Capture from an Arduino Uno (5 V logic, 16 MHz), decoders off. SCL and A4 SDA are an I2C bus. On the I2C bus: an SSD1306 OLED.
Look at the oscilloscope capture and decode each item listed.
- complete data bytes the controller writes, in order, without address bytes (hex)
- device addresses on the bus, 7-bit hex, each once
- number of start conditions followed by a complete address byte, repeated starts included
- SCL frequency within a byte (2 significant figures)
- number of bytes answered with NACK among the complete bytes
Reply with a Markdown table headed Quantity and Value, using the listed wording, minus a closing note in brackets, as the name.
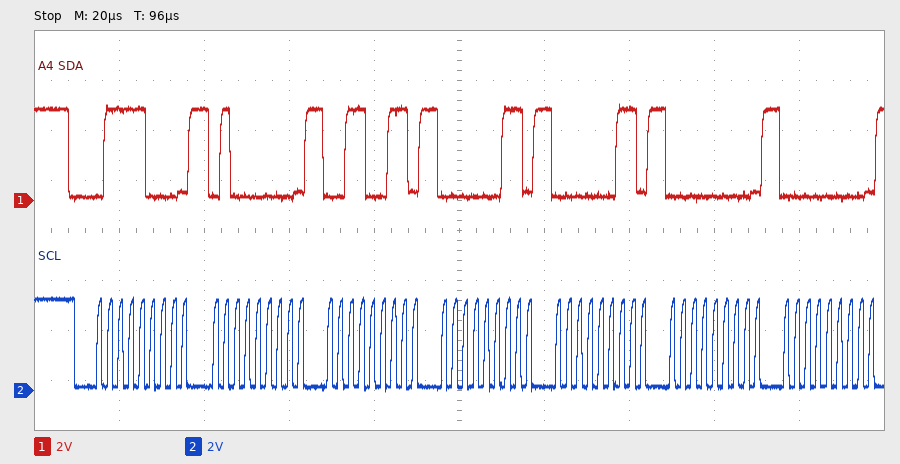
| Quantity | Value |
|---|---|
| complete data bytes the controller writes, in order, without address bytes | 40 33 03 03 00 00 |
| device addresses on the bus, 7-bit hex, each once | 0x3C |
| number of start conditions followed by a complete address byte, repeated starts included | 1 |
| SCL frequency within a byte | 400 kHz |
| number of bytes answered with NACK among the complete bytes | 0 |
